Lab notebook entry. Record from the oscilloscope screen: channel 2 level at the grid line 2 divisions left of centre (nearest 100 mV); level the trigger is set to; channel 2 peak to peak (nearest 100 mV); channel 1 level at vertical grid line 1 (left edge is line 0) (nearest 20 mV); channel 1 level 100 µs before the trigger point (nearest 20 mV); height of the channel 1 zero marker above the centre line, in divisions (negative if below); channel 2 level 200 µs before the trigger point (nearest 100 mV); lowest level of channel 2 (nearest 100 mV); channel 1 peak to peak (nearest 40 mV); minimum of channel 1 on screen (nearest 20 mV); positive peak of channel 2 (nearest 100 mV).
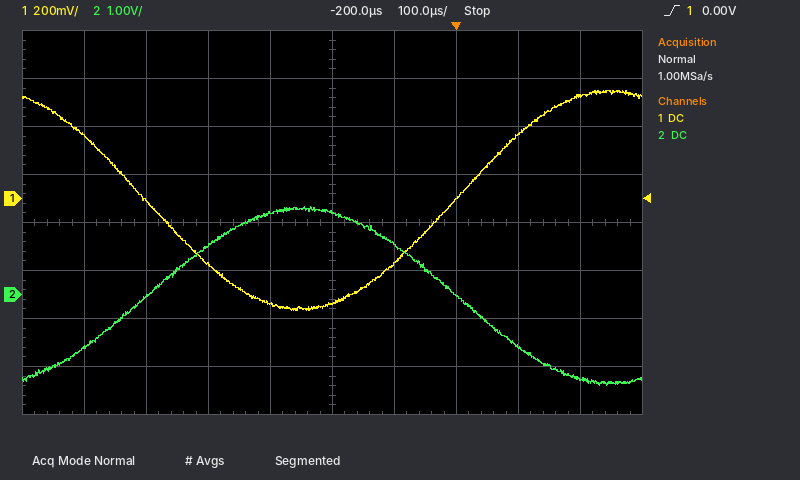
1.0 V
0.00 V
3.7 V
260 mV
-280 mV
+0.5 div
1.7 V
-1.9 V
920 mV
-460 mV
1.8 V
